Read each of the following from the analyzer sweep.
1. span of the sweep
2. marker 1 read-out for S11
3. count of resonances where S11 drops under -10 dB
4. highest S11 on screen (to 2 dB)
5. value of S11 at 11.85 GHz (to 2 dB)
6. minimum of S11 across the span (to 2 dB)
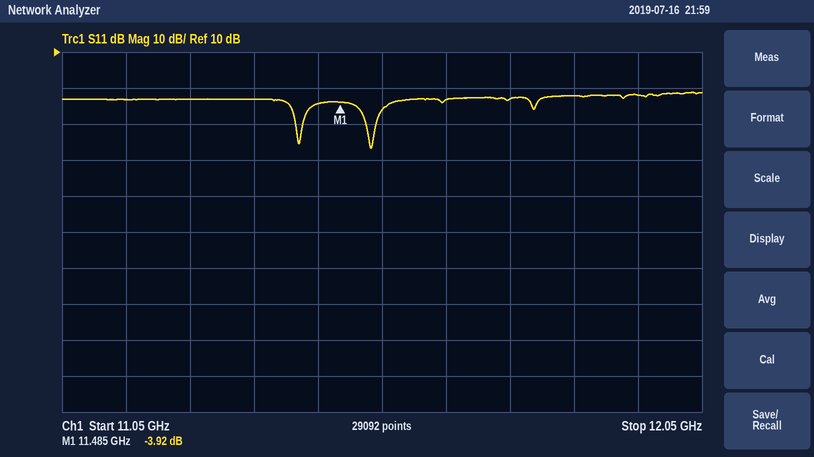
1 GHz
-3.92 dB
2
-2 dB
-2 dB
-16 dB
